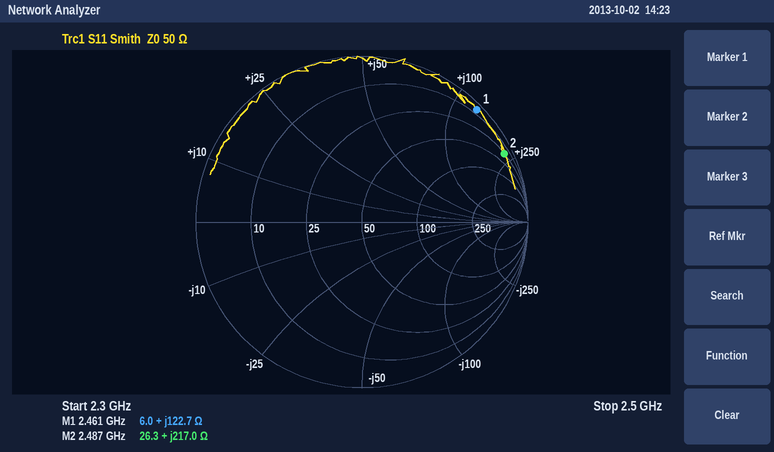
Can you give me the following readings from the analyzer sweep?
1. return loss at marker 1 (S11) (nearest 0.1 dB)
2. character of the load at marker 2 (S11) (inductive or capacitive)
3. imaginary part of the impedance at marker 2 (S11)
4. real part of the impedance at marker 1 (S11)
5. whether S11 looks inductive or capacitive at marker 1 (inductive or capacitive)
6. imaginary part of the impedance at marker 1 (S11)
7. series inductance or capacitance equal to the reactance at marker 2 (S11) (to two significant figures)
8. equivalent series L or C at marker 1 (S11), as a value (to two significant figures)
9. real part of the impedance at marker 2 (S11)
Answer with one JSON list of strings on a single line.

["0.3 dB", "inductive", "+217.0 Ω", "6.0 Ω", "inductive", "+122.7 Ω", "14 nH", "7.9 nH", "26.3 Ω"]
